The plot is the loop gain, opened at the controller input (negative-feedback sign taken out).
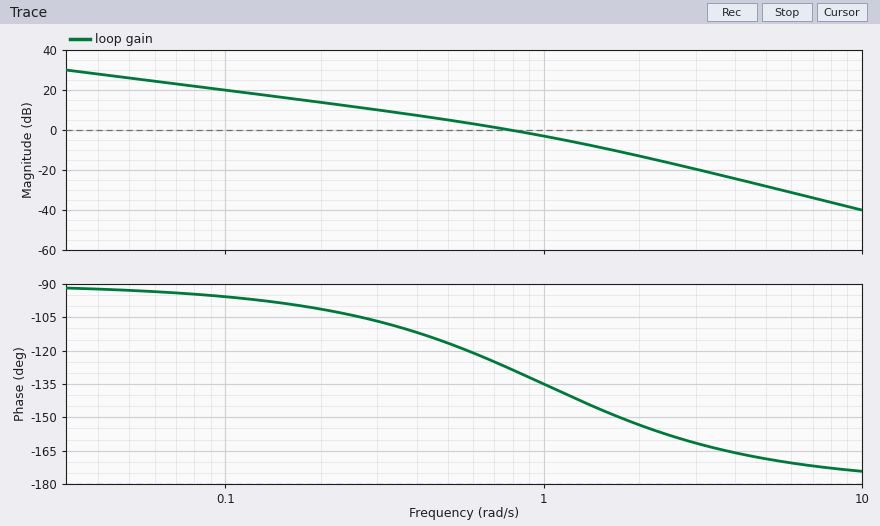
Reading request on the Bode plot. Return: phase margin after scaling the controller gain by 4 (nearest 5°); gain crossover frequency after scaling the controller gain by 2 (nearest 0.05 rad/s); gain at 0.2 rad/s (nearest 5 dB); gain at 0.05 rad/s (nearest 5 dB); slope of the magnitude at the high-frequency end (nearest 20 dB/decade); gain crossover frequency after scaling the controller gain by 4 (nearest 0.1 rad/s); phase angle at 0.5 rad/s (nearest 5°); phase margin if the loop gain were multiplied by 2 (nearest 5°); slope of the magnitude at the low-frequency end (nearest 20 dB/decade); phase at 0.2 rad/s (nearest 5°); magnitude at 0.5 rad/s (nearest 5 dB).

30°
1.25 rad/s
15 dB
25 dB
-40 dB/decade
1.9 rad/s
-115°
40°
-20 dB/decade
-100°
5 dB
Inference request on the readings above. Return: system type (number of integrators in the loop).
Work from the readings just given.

1
